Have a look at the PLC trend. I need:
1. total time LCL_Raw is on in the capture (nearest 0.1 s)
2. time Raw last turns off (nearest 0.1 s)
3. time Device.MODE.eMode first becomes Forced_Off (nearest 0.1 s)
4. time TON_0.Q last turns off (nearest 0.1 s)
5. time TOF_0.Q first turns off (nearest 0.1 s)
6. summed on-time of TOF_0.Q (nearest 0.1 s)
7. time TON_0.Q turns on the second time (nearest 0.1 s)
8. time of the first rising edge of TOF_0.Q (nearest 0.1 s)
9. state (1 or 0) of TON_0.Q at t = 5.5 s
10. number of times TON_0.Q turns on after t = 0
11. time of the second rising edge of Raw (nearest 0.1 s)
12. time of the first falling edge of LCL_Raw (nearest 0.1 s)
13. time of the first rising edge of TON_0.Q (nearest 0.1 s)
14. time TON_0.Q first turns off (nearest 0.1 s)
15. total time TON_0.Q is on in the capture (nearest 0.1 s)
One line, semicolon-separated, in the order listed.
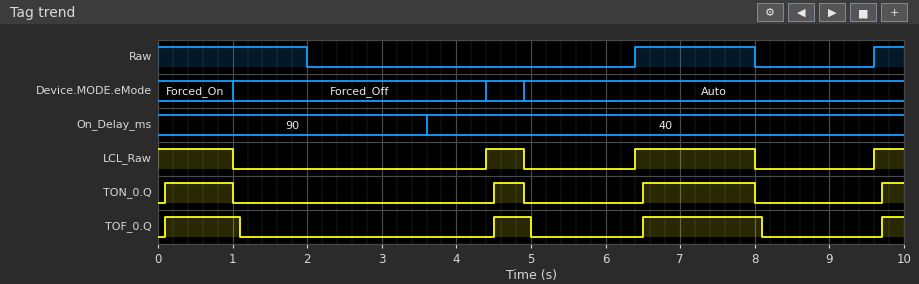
3.5 s; 8.0 s; 1.0 s; 8.0 s; 1.1 s; 3.4 s; 4.5 s; 0.1 s; 0; 4; 9.6 s; 1.0 s; 0.1 s; 1.0 s; 3.1 s
